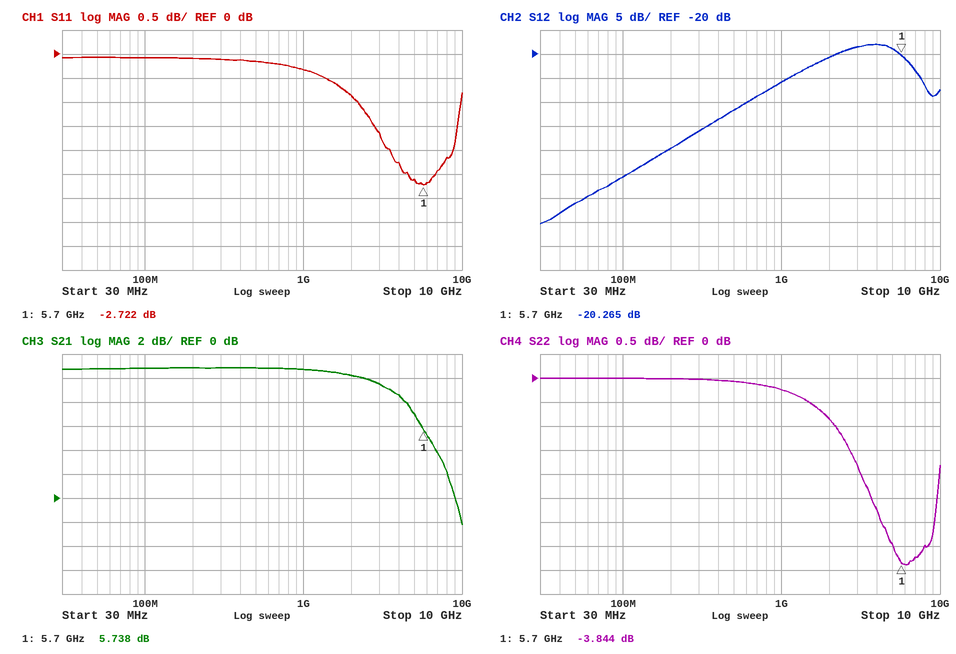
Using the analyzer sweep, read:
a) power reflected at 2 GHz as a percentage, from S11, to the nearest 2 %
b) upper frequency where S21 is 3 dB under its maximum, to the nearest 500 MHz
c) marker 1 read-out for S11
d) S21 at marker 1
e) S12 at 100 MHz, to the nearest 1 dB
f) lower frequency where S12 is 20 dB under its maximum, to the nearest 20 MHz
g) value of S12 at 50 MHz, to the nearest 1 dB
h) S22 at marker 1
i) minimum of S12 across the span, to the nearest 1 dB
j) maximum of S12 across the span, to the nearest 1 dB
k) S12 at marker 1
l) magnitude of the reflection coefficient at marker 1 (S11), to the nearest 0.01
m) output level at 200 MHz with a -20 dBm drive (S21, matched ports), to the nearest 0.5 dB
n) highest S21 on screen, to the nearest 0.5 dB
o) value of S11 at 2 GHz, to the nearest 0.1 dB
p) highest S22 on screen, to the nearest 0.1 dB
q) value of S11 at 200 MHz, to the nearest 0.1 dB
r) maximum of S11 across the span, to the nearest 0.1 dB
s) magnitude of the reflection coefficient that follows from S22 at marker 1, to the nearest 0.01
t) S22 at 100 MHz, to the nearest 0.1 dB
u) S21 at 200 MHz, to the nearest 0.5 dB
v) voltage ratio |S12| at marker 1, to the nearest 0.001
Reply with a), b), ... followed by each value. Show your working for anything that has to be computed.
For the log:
a) 10^(-0.9/10) ≈ 81.3 %, so 82 % to the nearest 2 %
b) 4.5 GHz
c) -2.722 dB
d) 5.738 dB
e) -46 dB
f) 240 MHz
g) -51 dB
h) -3.844 dB
i) -55 dB
j) -18 dB
k) -20.265 dB
l) 10^(-2.722/20) ≈ 0.73
m) -20 dBm + (11.0 dB) = -9.0 dBm
n) 11.0 dB
o) -0.9 dB
p) 0.0 dB
q) -0.1 dB
r) -0.1 dB
s) 10^(-3.844/20) ≈ 0.64
t) 0.0 dB
u) 11.0 dB
v) 10^(-20.265/20) ≈ 0.097
